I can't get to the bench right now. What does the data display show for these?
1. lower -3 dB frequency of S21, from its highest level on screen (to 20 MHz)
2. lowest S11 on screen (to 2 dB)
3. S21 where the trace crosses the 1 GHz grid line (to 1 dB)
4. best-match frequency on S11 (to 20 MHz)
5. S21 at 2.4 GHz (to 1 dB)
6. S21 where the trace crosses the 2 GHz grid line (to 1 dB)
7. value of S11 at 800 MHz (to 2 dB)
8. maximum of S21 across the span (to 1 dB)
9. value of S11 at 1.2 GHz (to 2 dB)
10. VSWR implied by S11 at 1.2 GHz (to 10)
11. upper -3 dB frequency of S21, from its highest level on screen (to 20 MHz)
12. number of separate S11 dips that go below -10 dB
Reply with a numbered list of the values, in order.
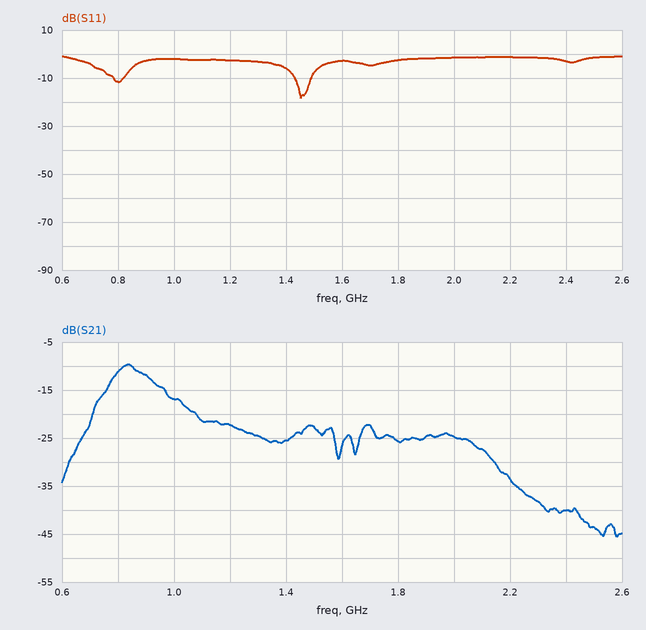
1. 780 MHz
2. -18 dB
3. -17 dB
4. 1.46 GHz
5. -40 dB
6. -25 dB
7. -12 dB
8. -10 dB
9. -2 dB
10. 10
11. 920 MHz
12. 2
